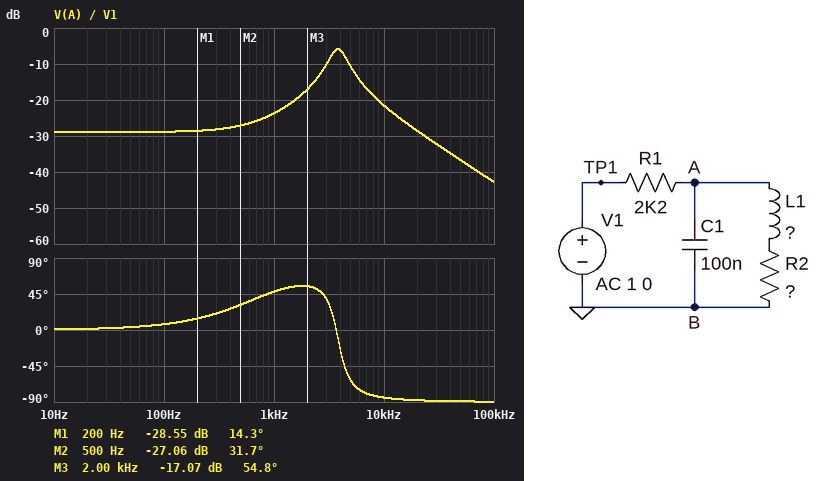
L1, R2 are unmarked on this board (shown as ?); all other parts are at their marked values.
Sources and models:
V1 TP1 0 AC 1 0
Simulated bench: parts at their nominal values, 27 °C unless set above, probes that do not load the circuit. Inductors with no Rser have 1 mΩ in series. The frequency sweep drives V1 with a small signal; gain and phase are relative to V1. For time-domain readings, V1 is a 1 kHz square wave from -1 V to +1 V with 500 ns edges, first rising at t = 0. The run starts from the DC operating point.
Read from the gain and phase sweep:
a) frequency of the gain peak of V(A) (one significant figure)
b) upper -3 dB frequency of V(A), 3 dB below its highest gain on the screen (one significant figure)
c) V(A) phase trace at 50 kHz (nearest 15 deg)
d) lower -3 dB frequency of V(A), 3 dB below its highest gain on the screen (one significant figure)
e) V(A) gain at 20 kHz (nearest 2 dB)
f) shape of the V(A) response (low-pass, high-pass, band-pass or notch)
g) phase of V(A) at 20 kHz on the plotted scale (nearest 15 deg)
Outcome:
4 kHz
5 kHz
-90 deg
3 kHz
-28 dB
band-pass
-90 deg
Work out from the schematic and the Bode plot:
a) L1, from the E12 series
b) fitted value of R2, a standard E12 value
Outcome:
18 mH
82 Ω
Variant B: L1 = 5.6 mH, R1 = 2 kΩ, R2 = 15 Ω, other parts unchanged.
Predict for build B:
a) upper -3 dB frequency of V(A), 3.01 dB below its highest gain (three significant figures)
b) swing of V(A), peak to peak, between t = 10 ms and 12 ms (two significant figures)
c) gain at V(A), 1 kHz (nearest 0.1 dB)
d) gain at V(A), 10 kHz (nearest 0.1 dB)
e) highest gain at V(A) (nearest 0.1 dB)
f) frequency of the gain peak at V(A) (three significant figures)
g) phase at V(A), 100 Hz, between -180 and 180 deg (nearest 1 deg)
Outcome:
7.39 kHz
460 mV
-34.2 dB
-16.9 dB
-3.7 dB
6.75 kHz
13 deg
